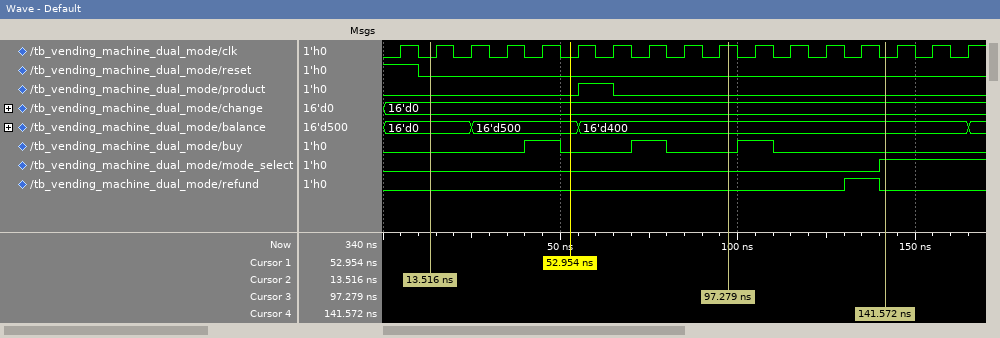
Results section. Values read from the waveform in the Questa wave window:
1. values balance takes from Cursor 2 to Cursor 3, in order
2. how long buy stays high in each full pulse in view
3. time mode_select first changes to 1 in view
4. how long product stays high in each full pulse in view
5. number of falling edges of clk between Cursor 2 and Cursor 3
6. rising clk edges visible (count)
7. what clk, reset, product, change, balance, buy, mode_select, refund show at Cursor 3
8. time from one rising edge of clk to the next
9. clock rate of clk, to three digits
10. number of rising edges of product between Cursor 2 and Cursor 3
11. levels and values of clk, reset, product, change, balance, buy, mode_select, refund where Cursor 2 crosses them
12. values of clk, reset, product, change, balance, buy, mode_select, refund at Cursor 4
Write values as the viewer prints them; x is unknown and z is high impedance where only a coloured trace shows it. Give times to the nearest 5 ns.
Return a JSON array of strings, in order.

["16'd0, 16'd500, 16'd400", "10 ns, 10 ns, 10 ns", "140 ns", "10 ns", "8", "17", "clk=1, reset=0, product=0, change=16'd0, balance=16'd400, buy=0, mode_select=0, refund=0", "10 ns", "100 MHz", "1", "clk=0, reset=0, product=0, change=16'd0, balance=16'd0, buy=0, mode_select=0, refund=0", "clk=0, reset=0, product=0, change=16'd0, balance=16'd400, buy=0, mode_select=1, refund=0"]
